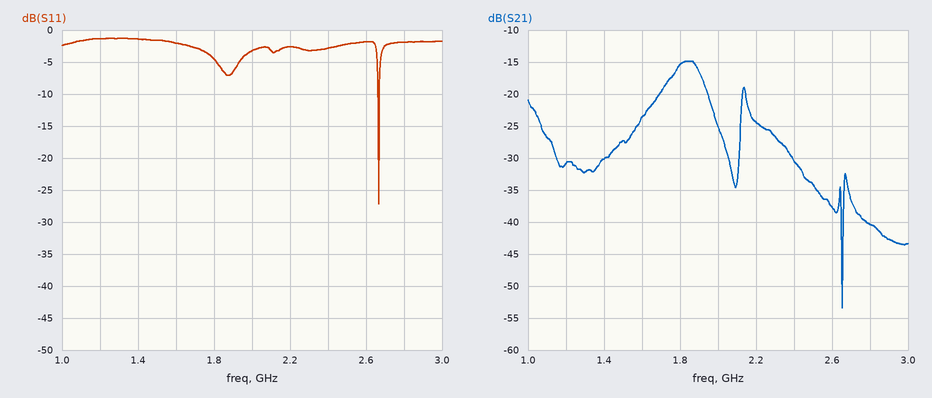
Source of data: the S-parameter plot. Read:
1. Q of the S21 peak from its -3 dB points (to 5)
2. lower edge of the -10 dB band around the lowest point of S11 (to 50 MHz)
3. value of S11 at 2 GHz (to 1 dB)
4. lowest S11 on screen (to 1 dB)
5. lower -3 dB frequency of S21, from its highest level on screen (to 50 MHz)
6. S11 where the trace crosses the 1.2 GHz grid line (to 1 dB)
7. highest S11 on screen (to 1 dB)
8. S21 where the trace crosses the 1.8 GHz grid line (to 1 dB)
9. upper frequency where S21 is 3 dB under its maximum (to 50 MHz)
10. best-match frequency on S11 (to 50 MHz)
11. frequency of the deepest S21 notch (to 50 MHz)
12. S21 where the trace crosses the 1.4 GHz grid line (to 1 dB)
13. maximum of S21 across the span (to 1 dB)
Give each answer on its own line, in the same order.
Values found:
10
2.65 GHz
-3 dB
-27 dB
1.75 GHz
-1 dB
-1 dB
-15 dB
1.90 GHz
2.65 GHz
2.65 GHz
-30 dB
-15 dB
